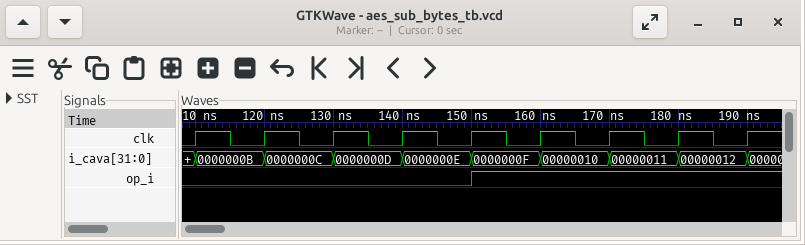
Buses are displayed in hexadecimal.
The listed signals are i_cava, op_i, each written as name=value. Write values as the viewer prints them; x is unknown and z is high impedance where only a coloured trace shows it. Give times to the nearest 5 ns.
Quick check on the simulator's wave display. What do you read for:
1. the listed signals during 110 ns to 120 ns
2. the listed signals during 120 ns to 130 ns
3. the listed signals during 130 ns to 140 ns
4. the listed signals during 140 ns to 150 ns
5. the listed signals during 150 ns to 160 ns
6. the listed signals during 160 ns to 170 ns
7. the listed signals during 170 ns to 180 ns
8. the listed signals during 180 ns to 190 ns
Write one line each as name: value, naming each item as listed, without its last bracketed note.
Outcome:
the listed signals during 110 ns to 120 ns: i_cava=0000000B, op_i=0
the listed signals during 120 ns to 130 ns: i_cava=0000000C, op_i=0
the listed signals during 130 ns to 140 ns: i_cava=0000000D, op_i=0
the listed signals during 140 ns to 150 ns: i_cava=0000000E, op_i=0
the listed signals during 150 ns to 160 ns: i_cava=0000000F, op_i=1
the listed signals during 160 ns to 170 ns: i_cava=00000010, op_i=1
the listed signals during 170 ns to 180 ns: i_cava=00000011, op_i=1
the listed signals during 180 ns to 190 ns: i_cava=00000012, op_i=1
